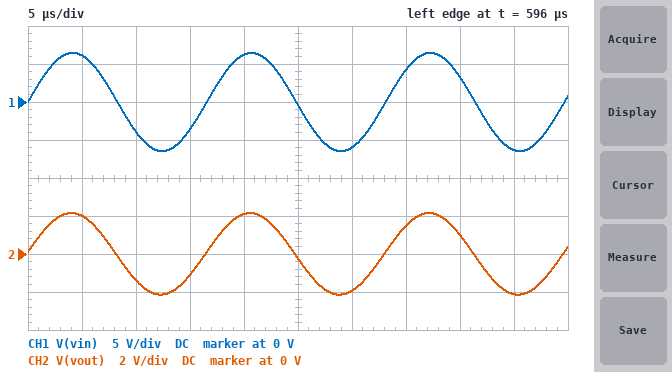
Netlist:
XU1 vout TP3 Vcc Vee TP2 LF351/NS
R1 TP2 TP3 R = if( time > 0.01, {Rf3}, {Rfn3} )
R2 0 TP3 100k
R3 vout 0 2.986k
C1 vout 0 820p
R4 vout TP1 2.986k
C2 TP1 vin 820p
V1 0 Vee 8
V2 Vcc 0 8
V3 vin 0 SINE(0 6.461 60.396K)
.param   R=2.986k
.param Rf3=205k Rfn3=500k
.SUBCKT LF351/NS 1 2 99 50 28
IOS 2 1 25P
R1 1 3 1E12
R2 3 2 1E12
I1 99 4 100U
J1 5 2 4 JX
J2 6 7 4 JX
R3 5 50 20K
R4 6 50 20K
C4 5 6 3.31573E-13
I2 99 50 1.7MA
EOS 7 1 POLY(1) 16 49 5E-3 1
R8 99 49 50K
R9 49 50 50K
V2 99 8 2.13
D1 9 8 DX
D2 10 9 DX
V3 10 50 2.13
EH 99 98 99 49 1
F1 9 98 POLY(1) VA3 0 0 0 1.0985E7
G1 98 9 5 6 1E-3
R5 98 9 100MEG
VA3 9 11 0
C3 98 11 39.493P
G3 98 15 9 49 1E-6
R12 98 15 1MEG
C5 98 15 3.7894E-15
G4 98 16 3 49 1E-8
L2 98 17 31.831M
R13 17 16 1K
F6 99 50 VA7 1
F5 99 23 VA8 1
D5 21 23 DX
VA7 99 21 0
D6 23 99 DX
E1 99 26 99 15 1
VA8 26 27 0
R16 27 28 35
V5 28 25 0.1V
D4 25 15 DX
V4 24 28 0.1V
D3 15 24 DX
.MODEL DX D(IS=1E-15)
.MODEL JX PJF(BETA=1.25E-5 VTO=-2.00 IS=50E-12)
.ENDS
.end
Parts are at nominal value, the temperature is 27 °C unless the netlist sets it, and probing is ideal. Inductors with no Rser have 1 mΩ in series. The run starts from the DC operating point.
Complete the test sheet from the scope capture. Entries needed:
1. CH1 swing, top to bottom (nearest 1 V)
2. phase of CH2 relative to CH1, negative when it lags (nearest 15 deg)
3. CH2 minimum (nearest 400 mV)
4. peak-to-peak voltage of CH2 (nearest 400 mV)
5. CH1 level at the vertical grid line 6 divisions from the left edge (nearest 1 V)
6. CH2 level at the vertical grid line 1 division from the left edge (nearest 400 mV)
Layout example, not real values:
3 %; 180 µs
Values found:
13 V; 0 deg; -2.0 V; 4.4 V; -6 V; 2.0 V
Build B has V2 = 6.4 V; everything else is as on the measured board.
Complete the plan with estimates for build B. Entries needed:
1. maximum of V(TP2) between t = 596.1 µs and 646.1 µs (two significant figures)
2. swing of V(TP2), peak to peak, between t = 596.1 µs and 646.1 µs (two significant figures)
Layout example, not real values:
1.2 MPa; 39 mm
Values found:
5.0 V; 12 V
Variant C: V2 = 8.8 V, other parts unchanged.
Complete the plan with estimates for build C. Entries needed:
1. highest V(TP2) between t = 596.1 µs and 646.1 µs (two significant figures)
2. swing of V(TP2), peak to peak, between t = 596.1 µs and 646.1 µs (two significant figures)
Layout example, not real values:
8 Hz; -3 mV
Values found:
7.4 V; 14 V
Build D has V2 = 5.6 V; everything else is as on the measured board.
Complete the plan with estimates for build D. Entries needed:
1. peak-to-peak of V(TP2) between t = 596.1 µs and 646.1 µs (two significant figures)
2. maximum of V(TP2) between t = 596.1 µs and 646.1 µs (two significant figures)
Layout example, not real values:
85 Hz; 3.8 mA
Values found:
11 V; 4.2 V
